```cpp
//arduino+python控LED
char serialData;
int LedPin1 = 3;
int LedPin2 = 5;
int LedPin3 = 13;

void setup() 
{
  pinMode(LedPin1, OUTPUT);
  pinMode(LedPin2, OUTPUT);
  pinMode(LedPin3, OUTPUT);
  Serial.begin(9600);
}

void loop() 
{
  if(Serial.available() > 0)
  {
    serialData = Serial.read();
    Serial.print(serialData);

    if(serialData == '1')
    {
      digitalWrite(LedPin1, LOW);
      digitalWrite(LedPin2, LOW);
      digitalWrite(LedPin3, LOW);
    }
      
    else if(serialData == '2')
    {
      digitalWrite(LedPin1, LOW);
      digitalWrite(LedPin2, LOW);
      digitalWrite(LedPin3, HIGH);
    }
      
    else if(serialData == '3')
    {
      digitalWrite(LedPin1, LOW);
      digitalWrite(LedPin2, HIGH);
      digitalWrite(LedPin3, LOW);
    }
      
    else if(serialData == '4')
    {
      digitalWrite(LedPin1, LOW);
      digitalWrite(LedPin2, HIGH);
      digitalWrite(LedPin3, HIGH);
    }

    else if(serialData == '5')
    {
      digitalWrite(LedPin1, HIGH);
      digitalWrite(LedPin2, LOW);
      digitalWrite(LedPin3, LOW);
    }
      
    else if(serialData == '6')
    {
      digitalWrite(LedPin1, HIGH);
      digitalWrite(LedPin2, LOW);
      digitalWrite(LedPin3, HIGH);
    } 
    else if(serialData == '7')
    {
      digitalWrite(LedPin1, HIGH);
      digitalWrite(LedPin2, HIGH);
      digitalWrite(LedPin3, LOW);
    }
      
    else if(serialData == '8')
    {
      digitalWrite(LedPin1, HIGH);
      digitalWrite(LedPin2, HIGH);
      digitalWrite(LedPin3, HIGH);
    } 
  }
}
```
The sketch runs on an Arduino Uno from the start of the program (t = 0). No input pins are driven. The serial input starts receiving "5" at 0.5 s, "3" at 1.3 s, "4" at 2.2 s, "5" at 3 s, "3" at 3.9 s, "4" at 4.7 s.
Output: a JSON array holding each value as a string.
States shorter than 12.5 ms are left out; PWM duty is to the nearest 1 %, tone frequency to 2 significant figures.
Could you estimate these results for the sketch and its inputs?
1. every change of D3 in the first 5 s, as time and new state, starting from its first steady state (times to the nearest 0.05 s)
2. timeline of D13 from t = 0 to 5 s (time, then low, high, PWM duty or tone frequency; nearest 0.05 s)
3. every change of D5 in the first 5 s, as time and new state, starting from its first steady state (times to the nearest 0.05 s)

["0 s low; 0.5 s high; 1.3 s low; 3 s high; 3.9 s low", "0 s low; 2.2 s high; 3 s low; 4.7 s high", "0 s low; 1.3 s high; 3 s low; 3.9 s high"]
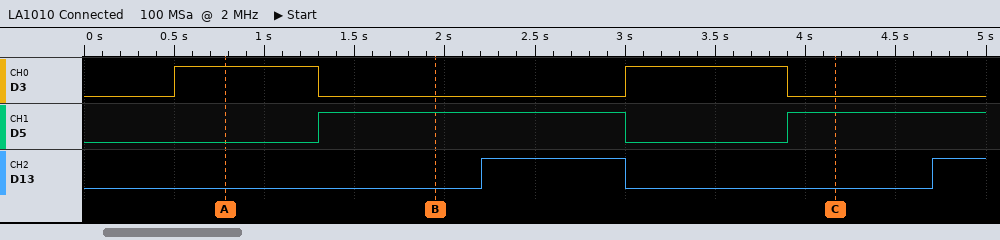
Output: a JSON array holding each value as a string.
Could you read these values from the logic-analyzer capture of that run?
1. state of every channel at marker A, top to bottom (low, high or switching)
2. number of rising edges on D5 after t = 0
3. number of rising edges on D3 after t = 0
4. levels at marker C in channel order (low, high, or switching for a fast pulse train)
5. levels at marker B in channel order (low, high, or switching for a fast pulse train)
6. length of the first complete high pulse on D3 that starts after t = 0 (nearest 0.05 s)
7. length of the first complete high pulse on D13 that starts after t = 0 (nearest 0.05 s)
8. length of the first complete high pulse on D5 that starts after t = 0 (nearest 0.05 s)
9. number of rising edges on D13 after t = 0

["D3 high, D5 low, D13 low", "2", "2", "D3 low, D5 high, D13 low", "D3 low, D5 high, D13 low", "0.80 s", "0.80 s", "1.70 s", "2"]
